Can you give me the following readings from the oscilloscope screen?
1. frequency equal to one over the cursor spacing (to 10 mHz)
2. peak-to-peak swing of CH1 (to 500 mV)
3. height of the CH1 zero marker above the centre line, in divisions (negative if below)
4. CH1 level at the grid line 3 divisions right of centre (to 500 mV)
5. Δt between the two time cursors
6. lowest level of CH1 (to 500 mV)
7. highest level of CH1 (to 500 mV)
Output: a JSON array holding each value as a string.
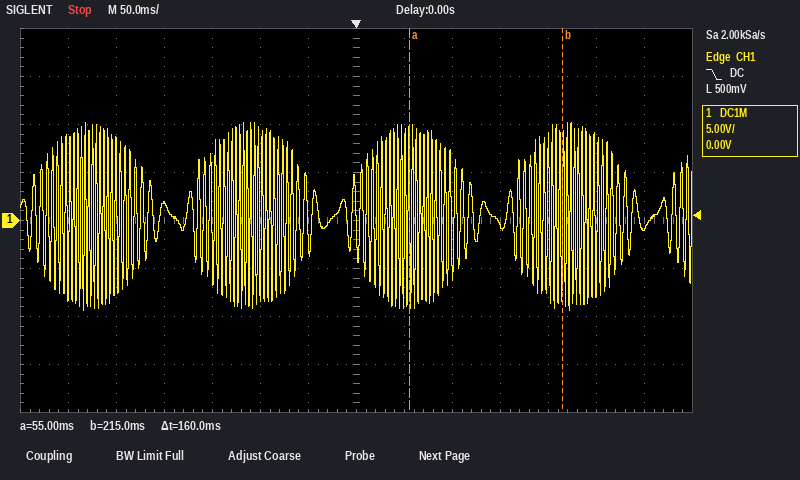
["6.25 Hz", "19.5 V", "0.0 div", "-500 mV", "160 ms", "-9.5 V", "10.0 V"]
